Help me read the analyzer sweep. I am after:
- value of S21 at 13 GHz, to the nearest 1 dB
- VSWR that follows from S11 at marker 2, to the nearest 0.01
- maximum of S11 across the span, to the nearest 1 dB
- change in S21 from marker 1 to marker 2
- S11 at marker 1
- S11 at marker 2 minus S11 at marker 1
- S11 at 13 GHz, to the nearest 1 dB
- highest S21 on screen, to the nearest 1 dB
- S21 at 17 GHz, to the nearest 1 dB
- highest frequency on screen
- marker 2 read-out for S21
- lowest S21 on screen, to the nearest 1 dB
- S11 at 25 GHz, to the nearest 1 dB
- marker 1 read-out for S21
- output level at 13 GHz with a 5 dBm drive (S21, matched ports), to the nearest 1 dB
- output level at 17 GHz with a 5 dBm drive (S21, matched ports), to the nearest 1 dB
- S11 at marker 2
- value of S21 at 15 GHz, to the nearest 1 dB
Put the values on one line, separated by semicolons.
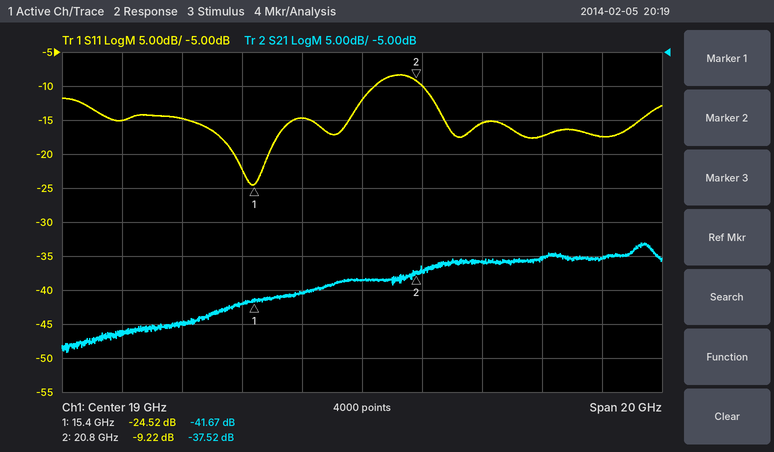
-45 dB; 2.06; -8 dB; 4.15 dB; -24.52 dB; 15.30 dB; -15 dB; -33 dB; -40 dB; 29 GHz; -37.52 dB; -49 dB; -17 dB; -41.67 dB; -40 dBm; -35 dBm; -9.22 dB; -42 dB
